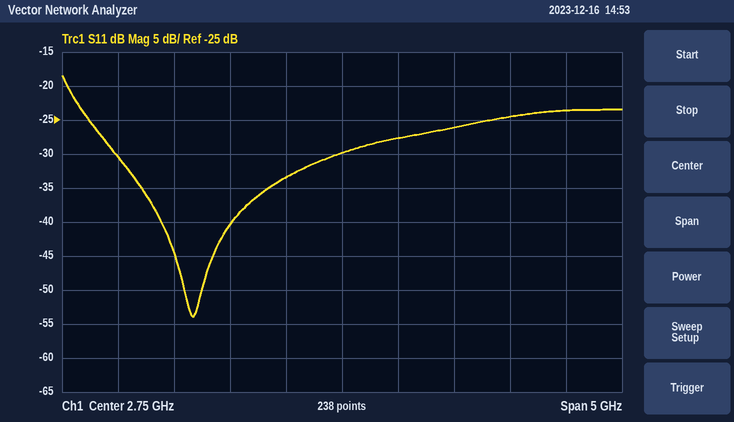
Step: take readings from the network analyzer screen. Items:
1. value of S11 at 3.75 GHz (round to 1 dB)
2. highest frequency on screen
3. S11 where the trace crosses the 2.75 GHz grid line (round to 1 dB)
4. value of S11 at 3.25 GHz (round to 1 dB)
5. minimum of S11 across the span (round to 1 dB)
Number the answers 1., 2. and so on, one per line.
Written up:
1. -26 dB
2. 5.25 GHz
3. -30 dB
4. -28 dB
5. -54 dB
